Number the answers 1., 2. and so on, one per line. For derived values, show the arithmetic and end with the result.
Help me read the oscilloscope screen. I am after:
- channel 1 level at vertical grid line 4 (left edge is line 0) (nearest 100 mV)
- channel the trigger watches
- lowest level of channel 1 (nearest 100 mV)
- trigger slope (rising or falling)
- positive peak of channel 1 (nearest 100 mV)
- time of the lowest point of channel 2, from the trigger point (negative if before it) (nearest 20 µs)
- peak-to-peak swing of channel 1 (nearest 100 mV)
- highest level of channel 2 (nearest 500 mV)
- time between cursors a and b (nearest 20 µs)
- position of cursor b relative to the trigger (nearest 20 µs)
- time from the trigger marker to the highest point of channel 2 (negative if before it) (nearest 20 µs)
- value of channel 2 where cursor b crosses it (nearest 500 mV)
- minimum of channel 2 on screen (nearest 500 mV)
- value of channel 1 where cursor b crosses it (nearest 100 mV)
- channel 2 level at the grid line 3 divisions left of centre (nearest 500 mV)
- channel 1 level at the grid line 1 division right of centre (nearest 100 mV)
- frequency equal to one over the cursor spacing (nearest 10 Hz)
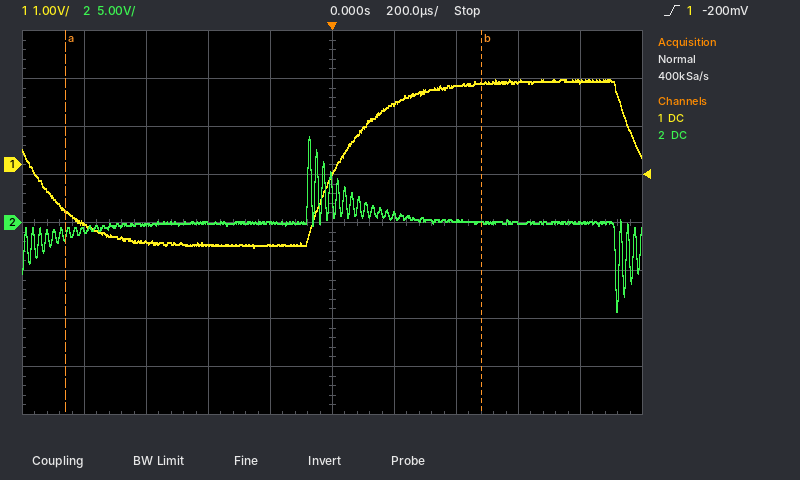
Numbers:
1. -1.7 V
2. channel 1
3. -1.7 V
4. rising
5. 1.8 V
6. +920 µs
7. 1.8 V − (-1.7 V) = 3.5 V
8. 9.0 V
9. 1.34 ms
10. +480 µs
11. -80 µs
12. 0.0 V
13. -9.5 V
14. 1.7 V
15. 0.0 V
16. 1.3 V
17. 1 / 1.34 ms ≈ 750 Hz
